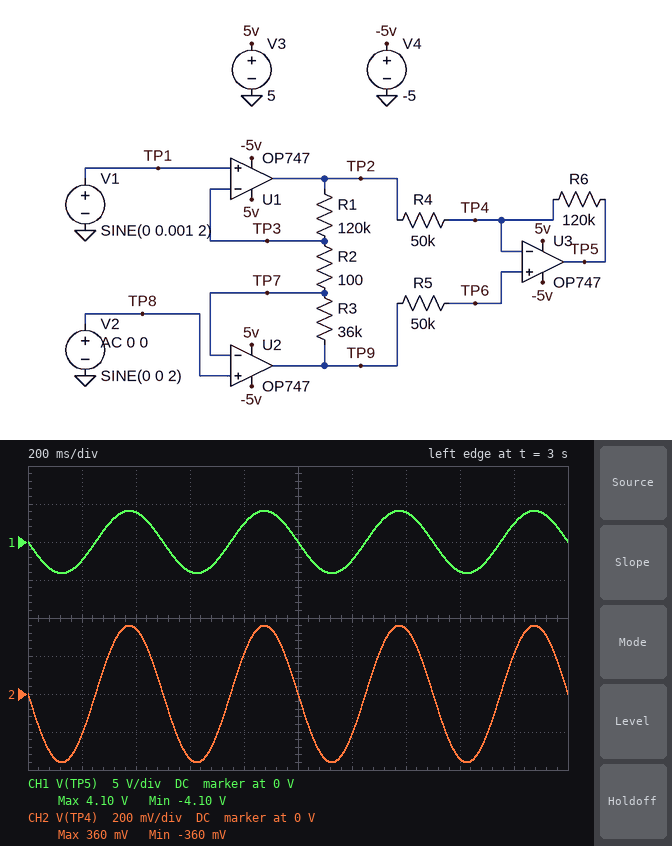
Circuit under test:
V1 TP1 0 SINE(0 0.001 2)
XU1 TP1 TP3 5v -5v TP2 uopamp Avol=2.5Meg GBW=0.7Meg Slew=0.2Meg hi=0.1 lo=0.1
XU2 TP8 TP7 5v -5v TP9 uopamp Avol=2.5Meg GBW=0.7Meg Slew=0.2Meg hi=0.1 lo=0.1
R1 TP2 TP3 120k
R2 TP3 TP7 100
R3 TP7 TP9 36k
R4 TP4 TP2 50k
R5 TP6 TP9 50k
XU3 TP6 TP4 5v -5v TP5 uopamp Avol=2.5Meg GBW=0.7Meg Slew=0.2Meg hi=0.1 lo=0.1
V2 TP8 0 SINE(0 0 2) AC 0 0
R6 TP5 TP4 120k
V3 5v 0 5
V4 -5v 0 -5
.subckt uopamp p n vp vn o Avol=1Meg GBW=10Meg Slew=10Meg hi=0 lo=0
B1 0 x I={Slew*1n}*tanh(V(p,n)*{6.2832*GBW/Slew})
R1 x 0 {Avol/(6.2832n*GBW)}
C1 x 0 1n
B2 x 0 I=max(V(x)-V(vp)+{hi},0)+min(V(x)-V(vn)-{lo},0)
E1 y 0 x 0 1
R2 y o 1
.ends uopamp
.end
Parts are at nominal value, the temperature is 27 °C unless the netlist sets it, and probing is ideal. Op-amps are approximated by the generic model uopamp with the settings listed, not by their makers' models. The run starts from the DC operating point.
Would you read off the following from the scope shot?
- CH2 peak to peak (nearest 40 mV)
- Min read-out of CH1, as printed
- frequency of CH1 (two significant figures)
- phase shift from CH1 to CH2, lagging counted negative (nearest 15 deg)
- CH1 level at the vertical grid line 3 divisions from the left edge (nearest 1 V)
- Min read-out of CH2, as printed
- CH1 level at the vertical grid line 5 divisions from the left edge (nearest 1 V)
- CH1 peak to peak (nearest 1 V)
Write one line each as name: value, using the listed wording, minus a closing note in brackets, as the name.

CH2 peak to peak: 720 mV
Min read-out of CH1, as printed: -4.10 V
frequency of CH1: 2.0 Hz
phase shift from CH1 to CH2, lagging counted negative: 0 deg
CH1 level at the vertical grid line 3 divisions from the left edge: -4 V
Min read-out of CH2, as printed: -360 mV
CH1 level at the vertical grid line 5 divisions from the left edge: 0 V
CH1 peak to peak: 8 V
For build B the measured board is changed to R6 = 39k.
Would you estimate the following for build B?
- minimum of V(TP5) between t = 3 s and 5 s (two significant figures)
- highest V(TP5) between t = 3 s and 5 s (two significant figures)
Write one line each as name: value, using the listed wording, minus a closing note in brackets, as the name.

minimum of V(TP5) between t = 3 s and 5 s: -1.6 V
highest V(TP5) between t = 3 s and 5 s: 1.6 V
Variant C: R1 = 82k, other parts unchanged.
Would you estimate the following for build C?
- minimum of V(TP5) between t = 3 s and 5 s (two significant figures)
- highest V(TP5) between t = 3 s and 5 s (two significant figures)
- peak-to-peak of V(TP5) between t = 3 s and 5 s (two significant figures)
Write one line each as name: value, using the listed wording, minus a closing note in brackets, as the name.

minimum of V(TP5) between t = 3 s and 5 s: -3.2 V
highest V(TP5) between t = 3 s and 5 s: 3.2 V
peak-to-peak of V(TP5) between t = 3 s and 5 s: 6.4 V
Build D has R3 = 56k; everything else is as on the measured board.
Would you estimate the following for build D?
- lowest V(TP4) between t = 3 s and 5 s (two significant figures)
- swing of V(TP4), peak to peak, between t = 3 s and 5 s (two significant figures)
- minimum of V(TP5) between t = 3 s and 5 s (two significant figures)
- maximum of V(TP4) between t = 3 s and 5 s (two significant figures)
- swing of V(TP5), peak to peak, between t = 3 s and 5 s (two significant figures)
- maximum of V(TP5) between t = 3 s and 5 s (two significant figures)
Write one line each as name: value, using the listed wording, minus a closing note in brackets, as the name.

lowest V(TP4) between t = 3 s and 5 s: -560 mV
swing of V(TP4), peak to peak, between t = 3 s and 5 s: 1.1 V
minimum of V(TP5) between t = 3 s and 5 s: -4.8 V
maximum of V(TP4) between t = 3 s and 5 s: 560 mV
swing of V(TP5), peak to peak, between t = 3 s and 5 s: 9.6 V
maximum of V(TP5) between t = 3 s and 5 s: 4.8 V
